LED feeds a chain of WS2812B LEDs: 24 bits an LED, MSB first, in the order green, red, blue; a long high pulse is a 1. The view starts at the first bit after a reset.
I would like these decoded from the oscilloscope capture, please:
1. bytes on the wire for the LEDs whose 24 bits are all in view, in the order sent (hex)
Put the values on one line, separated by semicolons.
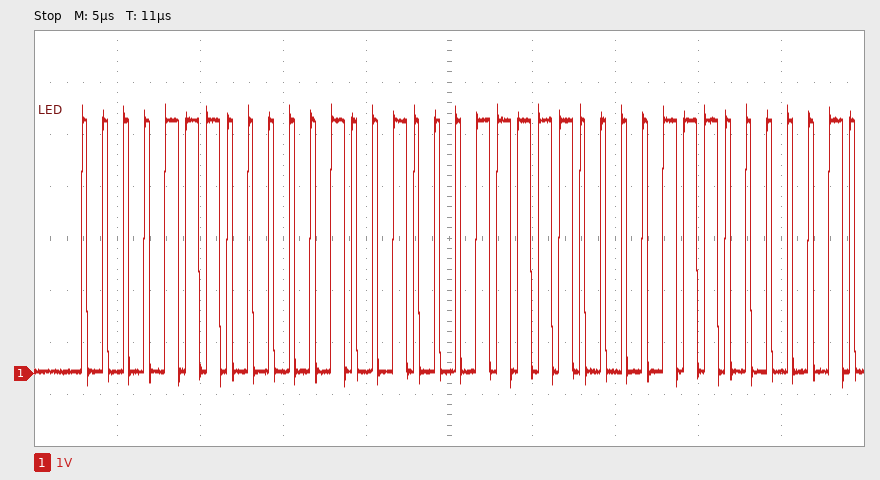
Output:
0E 09 1F
